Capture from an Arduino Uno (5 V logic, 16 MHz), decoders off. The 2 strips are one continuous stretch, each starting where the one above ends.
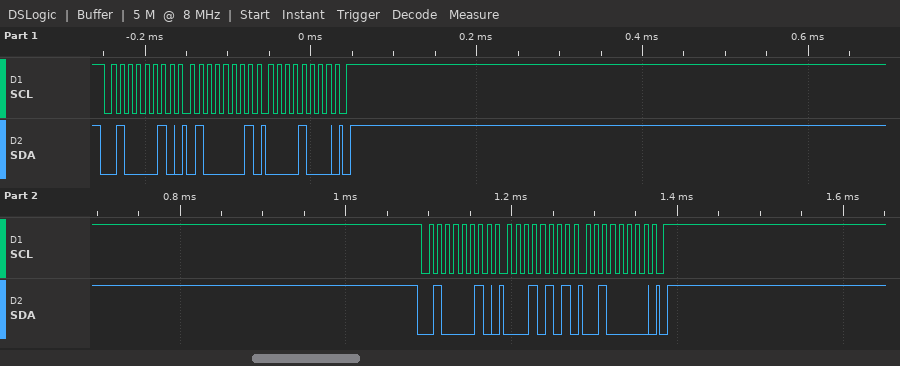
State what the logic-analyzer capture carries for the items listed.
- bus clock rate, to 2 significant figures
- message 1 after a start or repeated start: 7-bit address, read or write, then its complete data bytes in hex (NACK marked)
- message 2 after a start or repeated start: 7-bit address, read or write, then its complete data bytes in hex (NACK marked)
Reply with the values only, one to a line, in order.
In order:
100 kHz
0x21 write: 41 08
0x21 write: 15 20
